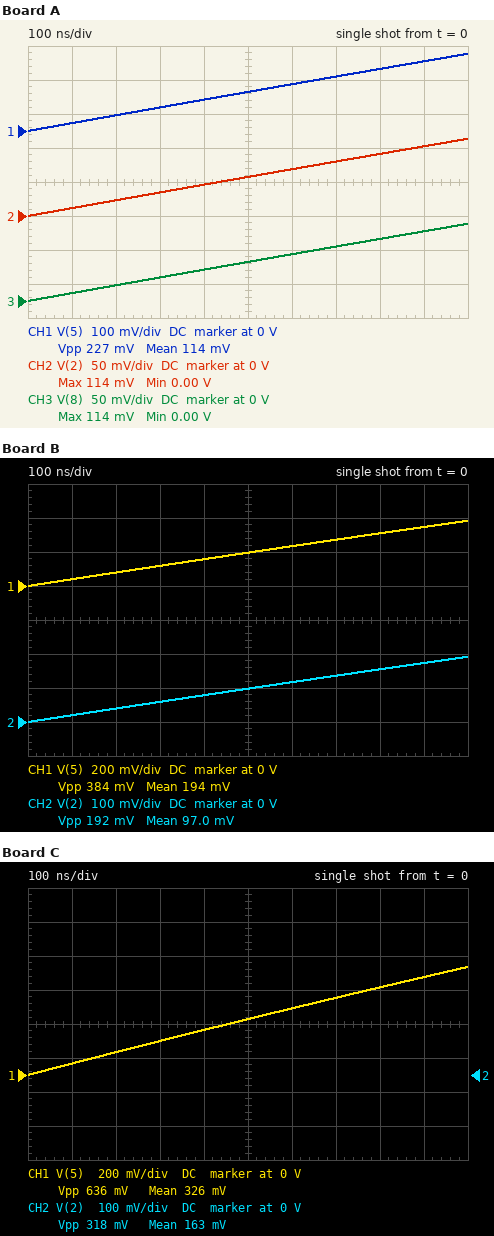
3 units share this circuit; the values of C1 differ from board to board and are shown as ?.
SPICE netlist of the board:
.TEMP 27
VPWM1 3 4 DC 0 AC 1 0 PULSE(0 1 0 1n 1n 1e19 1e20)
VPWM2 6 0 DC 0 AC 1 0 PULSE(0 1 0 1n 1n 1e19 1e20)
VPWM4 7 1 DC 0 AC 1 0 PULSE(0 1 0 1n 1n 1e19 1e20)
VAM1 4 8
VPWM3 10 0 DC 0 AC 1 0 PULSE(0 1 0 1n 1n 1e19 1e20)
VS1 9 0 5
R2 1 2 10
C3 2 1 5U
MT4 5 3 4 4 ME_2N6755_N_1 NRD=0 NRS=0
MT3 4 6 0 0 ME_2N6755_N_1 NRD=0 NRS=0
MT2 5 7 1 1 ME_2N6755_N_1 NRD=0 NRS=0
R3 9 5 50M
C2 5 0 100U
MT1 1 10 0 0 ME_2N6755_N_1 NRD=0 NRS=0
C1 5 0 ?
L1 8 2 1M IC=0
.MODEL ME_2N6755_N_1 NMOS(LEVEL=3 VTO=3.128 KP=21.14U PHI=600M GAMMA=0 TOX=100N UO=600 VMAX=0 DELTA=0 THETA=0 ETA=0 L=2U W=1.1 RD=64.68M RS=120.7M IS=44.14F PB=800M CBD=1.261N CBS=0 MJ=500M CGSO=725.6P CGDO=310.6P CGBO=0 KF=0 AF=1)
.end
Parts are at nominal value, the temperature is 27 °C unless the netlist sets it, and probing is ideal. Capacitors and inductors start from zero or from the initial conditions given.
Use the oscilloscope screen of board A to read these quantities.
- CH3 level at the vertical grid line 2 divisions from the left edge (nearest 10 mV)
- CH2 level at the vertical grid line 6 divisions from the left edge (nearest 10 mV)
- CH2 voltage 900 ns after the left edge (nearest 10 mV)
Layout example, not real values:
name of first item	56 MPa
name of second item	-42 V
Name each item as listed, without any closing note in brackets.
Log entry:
CH3 level at the vertical grid line 2 divisions from the left edge	20 mV
CH2 level at the vertical grid line 6 divisions from the left edge	70 mV
CH2 voltage 900 ns after the left edge	100 mV
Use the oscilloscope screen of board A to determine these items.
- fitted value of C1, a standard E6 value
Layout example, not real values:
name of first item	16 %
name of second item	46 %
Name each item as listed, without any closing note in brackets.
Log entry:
fitted value of C1, a standard E6 value	330 µF
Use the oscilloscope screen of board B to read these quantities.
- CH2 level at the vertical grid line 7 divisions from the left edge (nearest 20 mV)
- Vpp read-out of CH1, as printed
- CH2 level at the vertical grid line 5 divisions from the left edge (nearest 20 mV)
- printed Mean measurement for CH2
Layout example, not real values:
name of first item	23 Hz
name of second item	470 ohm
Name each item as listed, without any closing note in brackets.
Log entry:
CH2 level at the vertical grid line 7 divisions from the left edge	140 mV
Vpp read-out of CH1, as printed	384 mV
CH2 level at the vertical grid line 5 divisions from the left edge	100 mV
printed Mean measurement for CH2	97.0 mV
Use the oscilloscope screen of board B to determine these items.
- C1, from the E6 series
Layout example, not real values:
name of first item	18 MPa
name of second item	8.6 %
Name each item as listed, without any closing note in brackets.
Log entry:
C1, from the E6 series	150 µF
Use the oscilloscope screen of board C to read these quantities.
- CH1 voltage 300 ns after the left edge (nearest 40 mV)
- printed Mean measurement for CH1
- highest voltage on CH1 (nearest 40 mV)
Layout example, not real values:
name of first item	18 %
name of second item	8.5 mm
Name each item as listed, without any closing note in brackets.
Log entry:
CH1 voltage 300 ns after the left edge	200 mV
printed Mean measurement for CH1	326 mV
highest voltage on CH1	640 mV
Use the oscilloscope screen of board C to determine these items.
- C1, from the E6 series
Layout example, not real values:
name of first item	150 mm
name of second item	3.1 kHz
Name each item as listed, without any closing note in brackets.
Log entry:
C1, from the E6 series	47 µF
